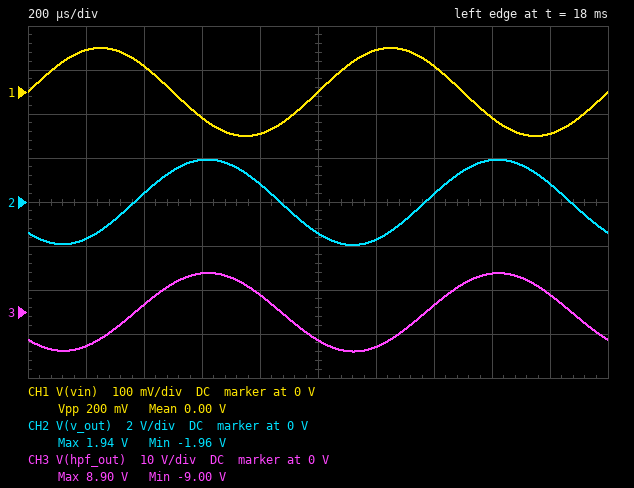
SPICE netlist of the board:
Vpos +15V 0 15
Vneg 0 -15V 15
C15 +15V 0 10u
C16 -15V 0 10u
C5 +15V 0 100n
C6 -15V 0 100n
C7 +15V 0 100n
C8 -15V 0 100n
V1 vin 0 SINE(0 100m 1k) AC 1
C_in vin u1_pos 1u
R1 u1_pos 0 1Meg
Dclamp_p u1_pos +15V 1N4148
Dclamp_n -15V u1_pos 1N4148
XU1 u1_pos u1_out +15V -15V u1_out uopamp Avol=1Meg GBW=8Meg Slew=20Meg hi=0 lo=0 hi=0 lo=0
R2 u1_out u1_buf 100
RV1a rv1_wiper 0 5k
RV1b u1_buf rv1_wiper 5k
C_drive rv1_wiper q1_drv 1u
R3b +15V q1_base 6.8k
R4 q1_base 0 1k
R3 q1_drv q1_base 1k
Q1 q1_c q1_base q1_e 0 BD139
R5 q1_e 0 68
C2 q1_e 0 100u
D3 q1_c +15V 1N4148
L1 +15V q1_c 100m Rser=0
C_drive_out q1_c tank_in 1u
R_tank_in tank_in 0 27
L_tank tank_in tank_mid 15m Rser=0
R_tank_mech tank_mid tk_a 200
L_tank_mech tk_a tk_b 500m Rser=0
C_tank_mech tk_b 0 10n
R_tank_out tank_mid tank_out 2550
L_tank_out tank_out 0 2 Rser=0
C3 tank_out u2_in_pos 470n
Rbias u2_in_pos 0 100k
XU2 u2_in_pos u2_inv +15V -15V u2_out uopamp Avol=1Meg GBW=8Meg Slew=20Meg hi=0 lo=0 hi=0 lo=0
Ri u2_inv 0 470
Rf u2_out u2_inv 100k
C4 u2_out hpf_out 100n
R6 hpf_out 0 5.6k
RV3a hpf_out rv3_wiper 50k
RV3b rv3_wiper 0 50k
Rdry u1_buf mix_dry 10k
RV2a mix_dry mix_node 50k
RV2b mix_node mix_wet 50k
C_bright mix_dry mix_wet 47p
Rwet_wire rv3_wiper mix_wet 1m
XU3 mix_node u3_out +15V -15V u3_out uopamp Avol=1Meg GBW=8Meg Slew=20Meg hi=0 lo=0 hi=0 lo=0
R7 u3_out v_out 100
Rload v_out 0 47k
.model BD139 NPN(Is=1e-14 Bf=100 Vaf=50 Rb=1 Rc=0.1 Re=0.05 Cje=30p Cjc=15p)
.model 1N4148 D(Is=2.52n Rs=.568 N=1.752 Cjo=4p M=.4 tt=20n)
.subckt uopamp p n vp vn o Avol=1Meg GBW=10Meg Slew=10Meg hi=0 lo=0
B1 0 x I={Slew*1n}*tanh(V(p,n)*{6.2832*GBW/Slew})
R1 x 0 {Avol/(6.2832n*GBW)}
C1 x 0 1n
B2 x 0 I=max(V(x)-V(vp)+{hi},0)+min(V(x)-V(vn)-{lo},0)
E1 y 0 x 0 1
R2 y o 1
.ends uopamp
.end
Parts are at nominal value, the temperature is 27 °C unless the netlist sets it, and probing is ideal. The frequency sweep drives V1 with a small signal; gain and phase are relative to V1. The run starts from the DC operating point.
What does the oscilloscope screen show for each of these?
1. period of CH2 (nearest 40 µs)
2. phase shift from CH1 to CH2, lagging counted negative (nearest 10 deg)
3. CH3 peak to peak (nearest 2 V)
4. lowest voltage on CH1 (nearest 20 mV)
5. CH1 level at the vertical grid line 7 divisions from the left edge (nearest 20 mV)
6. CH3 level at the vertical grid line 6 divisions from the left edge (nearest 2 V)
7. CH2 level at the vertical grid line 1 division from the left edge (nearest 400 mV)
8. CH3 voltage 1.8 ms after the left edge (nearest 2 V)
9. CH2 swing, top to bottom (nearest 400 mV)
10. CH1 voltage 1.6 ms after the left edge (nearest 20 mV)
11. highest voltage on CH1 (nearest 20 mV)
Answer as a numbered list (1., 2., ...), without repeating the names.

1. 1.00 ms
2. -130 deg
3. 18 V
4. -100 mV
5. 60 mV
6. -8 V
7. -1.6 V
8. 4 V
9. 4.0 V
10. -60 mV
11. 100 mV
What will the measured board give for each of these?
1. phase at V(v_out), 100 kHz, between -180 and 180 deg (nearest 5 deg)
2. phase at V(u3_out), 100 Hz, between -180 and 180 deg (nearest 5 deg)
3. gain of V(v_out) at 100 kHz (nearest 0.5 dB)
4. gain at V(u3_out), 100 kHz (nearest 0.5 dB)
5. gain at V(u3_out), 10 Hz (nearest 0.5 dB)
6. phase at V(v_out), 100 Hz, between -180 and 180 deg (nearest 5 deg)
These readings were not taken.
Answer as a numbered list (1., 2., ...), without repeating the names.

1. 85 deg
2. 0 deg
3. 14.0 dB
4. 14.0 dB
5. -5.0 dB
6. 0 deg
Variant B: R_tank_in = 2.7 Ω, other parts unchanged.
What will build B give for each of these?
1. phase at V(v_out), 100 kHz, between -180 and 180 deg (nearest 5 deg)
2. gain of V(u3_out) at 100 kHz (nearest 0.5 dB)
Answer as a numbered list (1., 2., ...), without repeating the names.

1. 45 deg
2. -2.0 dB
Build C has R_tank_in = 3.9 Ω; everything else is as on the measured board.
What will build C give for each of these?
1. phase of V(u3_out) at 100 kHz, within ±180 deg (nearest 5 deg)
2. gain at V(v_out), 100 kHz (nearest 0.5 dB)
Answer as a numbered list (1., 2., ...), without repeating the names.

1. 55 deg
2. -0.5 dB
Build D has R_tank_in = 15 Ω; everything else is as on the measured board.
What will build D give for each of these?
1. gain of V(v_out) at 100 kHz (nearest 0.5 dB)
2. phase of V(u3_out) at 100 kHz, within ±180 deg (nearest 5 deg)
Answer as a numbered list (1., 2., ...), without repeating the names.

1. 9.0 dB
2. 80 deg
